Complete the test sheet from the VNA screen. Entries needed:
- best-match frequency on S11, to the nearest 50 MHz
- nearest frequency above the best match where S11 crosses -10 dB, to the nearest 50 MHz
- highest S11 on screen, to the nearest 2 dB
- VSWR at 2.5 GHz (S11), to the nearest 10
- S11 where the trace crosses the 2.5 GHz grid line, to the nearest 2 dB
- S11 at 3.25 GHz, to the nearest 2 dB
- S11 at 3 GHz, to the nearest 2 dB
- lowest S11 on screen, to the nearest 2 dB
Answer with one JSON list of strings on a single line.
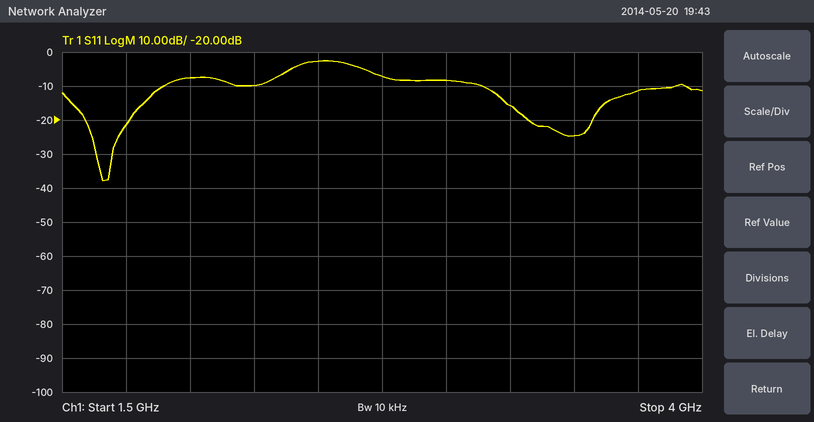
["1.65 GHz", "1.90 GHz", "-2 dB", "10", "-2 dB", "-16 dB", "-8 dB", "-38 dB"]
